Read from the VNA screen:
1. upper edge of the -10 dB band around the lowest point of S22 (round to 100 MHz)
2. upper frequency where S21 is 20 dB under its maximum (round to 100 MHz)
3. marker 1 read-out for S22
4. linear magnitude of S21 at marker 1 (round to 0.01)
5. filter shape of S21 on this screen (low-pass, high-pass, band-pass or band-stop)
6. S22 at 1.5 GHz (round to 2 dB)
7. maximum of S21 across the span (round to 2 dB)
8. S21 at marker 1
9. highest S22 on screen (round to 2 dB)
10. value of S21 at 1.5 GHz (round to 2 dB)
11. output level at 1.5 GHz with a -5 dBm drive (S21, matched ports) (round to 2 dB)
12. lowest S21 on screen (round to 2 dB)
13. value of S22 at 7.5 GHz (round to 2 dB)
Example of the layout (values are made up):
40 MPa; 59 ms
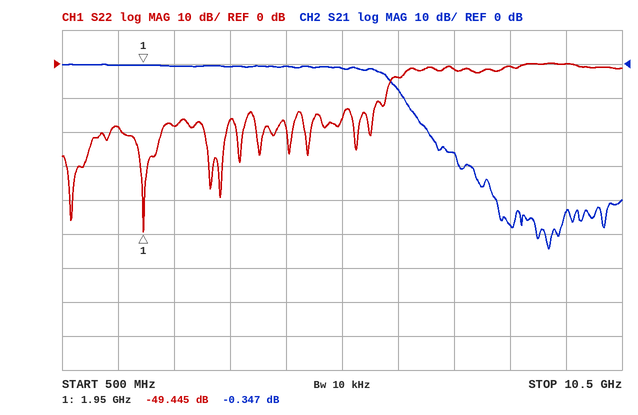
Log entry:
6.3 GHz; 7.0 GHz; -49.445 dB; 0.96; low-pass; -18 dB; 0 dB; -0.347 dB; 0 dB; 0 dB; -6 dBm; -54 dB; -2 dB
